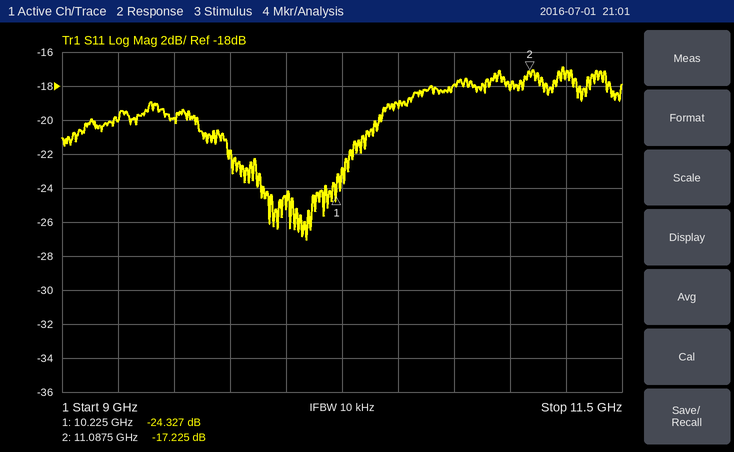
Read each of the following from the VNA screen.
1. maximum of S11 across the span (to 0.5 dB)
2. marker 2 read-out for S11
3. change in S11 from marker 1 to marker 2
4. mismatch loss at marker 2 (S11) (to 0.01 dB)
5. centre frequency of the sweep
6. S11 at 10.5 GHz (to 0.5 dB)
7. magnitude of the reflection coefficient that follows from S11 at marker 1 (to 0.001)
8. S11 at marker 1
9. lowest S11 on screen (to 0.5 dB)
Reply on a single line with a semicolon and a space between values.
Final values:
-17.0 dB; -17.225 dB; 7.102 dB; 0.08 dB; 10.25 GHz; -19.0 dB; 0.061; -24.327 dB; -27.0 dB
